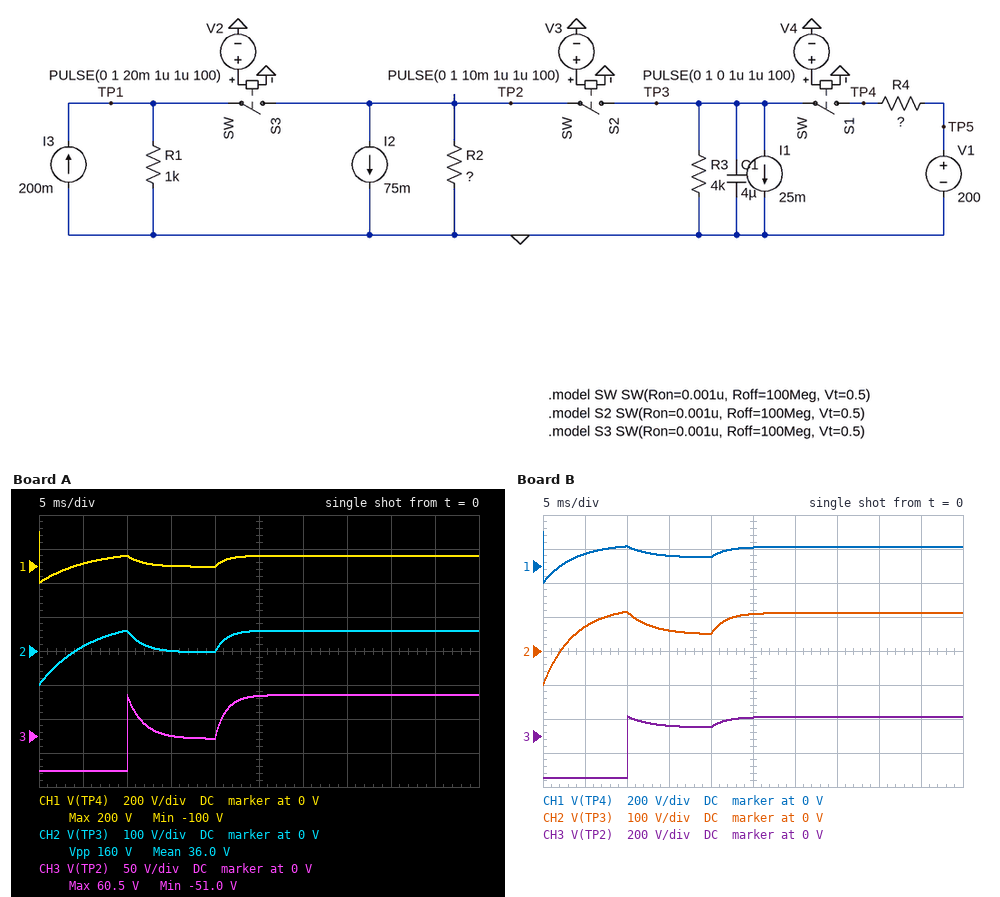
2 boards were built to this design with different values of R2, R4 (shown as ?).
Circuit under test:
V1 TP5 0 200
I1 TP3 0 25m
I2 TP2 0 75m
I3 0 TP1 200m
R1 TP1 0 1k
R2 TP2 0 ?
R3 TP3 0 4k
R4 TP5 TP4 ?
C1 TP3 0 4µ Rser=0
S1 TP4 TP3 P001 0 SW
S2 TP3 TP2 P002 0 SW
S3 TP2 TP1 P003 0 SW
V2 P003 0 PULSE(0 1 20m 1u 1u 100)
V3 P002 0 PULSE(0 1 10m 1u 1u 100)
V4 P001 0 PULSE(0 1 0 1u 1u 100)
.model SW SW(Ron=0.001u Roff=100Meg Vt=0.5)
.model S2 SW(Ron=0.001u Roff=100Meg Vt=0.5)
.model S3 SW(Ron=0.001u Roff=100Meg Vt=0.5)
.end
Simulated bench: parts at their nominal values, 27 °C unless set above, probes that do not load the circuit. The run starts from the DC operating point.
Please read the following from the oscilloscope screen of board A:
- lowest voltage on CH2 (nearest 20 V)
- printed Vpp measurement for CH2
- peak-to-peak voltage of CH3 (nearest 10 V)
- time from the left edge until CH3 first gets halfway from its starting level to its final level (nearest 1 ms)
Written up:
-100 V
160 V
110 V
10 ms
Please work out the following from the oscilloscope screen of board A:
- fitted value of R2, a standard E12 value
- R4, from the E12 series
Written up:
680 Ω
2.2 kΩ
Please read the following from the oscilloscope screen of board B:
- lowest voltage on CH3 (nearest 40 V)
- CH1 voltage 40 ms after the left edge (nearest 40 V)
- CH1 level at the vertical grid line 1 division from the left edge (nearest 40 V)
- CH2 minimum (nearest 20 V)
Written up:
-240 V
120 V
80 V
-100 V
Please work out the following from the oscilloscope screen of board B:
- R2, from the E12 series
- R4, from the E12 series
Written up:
3.3 kΩ
1.2 kΩ
